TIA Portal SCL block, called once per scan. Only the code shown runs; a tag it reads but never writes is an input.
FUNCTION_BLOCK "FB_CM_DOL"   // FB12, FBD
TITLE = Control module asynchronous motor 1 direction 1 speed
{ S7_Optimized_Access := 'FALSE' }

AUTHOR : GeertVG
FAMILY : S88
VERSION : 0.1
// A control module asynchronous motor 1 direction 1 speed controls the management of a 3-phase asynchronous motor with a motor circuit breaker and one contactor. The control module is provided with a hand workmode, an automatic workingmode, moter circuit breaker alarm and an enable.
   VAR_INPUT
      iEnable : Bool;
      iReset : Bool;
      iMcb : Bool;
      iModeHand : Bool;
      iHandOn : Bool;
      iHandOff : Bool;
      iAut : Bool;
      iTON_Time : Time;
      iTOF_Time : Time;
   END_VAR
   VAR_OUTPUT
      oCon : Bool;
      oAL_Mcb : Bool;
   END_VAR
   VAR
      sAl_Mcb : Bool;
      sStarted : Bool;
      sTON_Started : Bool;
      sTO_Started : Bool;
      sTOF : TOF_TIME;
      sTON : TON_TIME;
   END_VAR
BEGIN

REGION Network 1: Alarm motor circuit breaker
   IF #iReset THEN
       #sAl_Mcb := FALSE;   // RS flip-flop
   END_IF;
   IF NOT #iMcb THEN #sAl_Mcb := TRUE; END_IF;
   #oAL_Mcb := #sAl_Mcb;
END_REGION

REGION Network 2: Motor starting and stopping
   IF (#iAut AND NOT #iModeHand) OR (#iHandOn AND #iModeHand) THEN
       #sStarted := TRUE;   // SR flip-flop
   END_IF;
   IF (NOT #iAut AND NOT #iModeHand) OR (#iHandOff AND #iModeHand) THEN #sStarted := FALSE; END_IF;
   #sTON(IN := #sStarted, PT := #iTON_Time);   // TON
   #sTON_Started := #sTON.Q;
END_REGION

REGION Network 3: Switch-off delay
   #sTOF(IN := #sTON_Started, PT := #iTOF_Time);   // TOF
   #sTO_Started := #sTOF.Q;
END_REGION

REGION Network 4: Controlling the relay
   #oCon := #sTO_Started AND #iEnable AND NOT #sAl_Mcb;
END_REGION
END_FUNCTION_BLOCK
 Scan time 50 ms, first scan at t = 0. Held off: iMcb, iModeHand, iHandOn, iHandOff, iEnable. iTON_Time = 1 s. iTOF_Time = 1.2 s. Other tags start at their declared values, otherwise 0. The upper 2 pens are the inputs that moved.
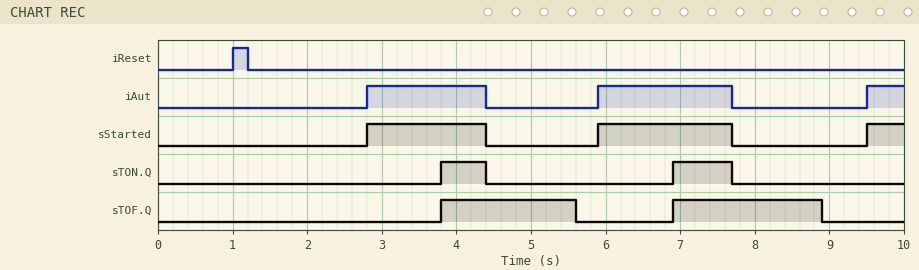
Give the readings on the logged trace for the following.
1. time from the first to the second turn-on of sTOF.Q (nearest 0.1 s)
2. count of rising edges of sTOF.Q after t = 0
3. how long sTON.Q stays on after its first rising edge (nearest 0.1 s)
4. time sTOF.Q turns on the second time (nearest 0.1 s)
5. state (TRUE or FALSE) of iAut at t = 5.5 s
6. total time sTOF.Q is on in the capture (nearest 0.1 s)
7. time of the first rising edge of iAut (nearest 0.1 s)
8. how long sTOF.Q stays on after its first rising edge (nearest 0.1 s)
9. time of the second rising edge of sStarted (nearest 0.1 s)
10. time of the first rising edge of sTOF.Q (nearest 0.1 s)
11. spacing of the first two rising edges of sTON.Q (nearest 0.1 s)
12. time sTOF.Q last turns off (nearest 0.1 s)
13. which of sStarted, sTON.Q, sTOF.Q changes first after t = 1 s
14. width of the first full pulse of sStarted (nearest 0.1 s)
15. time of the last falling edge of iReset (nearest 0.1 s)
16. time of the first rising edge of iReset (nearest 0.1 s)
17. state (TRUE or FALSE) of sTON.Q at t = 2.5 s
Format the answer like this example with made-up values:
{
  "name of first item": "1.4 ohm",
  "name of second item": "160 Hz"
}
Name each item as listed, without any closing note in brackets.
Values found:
{
  "time from the first to the second turn-on of sTOF.Q": "3.1 s",
  "count of rising edges of sTOF.Q after t = 0": "2",
  "how long sTON.Q stays on after its first rising edge": "0.6 s",
  "time sTOF.Q turns on the second time": "6.9 s",
  "state (TRUE or FALSE) of iAut at t = 5.5 s": "FALSE",
  "total time sTOF.Q is on in the capture": "3.8 s",
  "time of the first rising edge of iAut": "2.8 s",
  "how long sTOF.Q stays on after its first rising edge": "1.8 s",
  "time of the second rising edge of sStarted": "5.9 s",
  "time of the first rising edge of sTOF.Q": "3.8 s",
  "spacing of the first two rising edges of sTON.Q": "3.1 s",
  "time sTOF.Q last turns off": "8.9 s",
  "which of sStarted, sTON.Q, sTOF.Q changes first after t = 1 s": "sStarted",
  "width of the first full pulse of sStarted": "1.6 s",
  "time of the last falling edge of iReset": "1.2 s",
  "time of the first rising edge of iReset": "1.0 s",
  "state (TRUE or FALSE) of sTON.Q at t = 2.5 s": "FALSE"
}
